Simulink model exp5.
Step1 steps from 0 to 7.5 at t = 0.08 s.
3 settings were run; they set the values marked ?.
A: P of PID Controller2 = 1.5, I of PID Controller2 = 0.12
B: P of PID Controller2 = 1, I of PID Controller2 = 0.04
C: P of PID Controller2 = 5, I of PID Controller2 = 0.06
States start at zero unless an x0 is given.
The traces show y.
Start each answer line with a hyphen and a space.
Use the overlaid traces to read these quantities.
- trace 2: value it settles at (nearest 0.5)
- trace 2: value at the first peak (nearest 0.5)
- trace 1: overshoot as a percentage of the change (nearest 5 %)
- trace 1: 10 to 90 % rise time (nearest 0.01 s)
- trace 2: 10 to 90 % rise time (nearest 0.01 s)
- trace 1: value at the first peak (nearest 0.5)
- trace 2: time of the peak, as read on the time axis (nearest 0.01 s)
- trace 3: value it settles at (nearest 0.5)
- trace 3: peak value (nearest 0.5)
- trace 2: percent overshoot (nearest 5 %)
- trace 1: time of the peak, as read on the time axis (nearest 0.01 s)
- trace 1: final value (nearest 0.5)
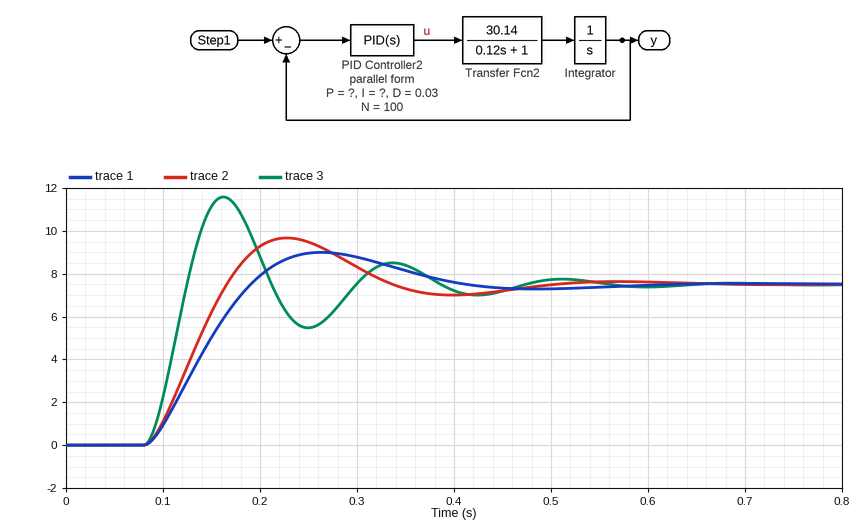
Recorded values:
- 7.5
- 9.5
- 20 %
- 0.08 s
- 0.06 s
- 9.0
- 0.23 s
- 7.5
- 11.5
- 30 %
- 0.26 s
- 7.5
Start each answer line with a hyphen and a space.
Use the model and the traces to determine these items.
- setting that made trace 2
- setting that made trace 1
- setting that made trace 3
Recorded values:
- A
- B
- C
